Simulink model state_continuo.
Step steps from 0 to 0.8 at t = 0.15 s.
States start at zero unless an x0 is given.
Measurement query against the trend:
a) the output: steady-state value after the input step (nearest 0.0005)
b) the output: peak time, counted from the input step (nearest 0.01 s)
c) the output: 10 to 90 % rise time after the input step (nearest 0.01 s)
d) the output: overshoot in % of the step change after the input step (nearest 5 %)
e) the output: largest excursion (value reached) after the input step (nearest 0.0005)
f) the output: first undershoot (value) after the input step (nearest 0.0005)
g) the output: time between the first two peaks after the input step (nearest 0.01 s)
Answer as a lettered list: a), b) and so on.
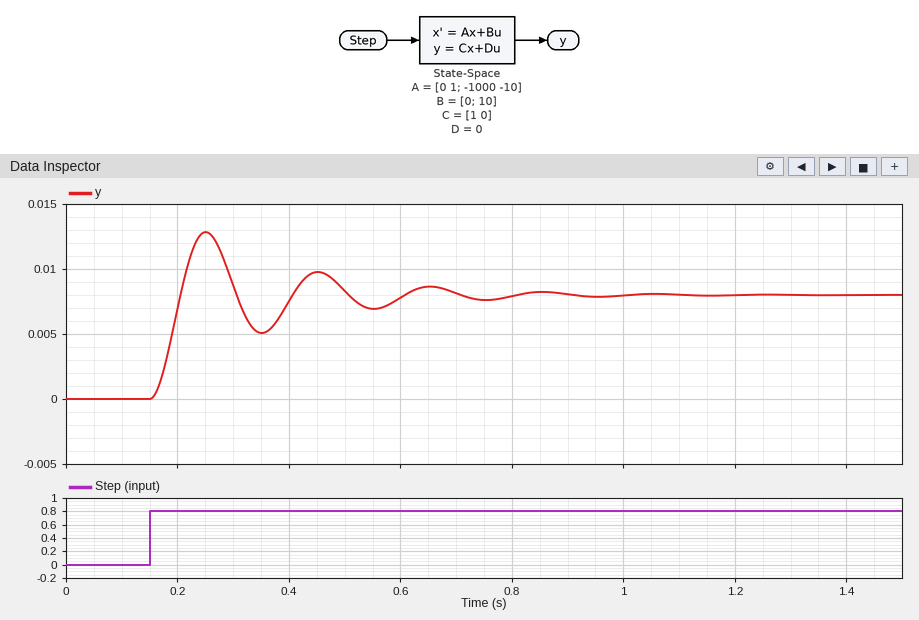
a) 0.0080
b) 0.10 s
c) 0.04 s
d) 60 %
e) 0.0130
f) 0.0050
g) 0.20 s
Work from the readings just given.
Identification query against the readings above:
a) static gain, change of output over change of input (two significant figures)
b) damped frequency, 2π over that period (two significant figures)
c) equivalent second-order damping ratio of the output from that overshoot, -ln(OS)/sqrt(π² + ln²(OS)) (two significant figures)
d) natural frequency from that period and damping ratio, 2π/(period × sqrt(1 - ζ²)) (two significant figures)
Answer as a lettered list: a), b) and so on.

a) 0.010
b) 31 rad/s
c) 0.16
d) 32 rad/s
